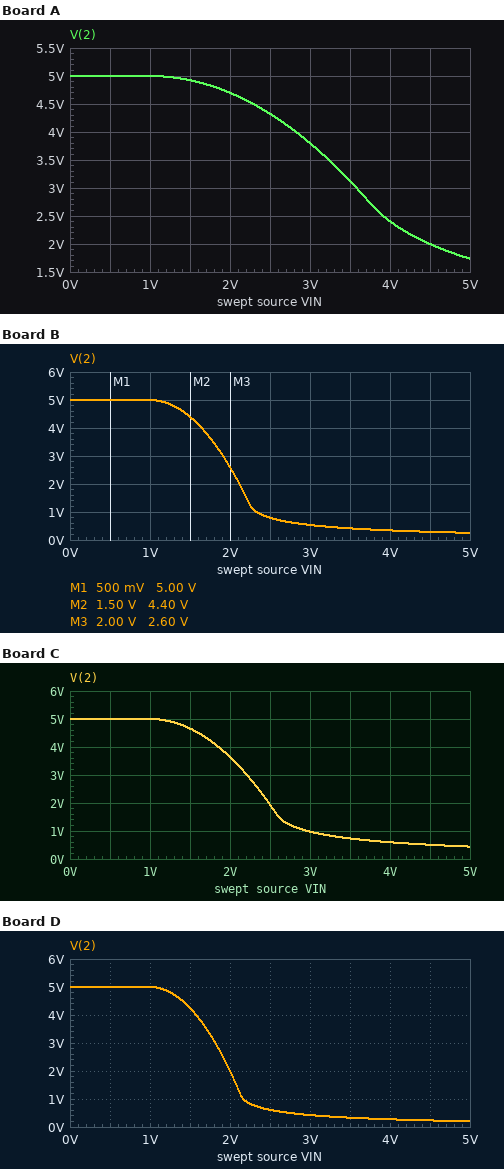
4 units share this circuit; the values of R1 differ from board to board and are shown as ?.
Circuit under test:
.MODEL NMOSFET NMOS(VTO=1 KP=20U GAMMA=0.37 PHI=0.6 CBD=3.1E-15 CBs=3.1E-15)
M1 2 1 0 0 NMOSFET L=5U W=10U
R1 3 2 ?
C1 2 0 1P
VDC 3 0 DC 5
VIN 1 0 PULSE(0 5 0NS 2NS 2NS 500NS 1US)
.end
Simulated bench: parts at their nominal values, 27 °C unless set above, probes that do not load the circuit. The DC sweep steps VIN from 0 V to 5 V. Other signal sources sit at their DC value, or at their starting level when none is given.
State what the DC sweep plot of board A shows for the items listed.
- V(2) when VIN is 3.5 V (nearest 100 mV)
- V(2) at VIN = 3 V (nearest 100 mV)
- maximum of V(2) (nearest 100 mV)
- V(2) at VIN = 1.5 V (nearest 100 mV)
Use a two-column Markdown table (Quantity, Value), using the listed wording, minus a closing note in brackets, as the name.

| Quantity | Value |
|---|---|
| V(2) when VIN is 3.5 V | 3.1 V |
| V(2) at VIN = 3 V | 3.8 V |
| maximum of V(2) | 5.0 V |
| V(2) at VIN = 1.5 V | 4.9 V |
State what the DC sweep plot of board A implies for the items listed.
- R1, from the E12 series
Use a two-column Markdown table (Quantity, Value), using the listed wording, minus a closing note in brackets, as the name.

| Quantity | Value |
|---|---|
| R1, from the E12 series | 15 kΩ |
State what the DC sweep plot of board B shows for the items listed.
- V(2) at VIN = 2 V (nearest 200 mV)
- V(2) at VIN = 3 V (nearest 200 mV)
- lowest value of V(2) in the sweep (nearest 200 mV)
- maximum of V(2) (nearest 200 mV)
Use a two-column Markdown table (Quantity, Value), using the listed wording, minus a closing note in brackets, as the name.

| Quantity | Value |
|---|---|
| V(2) at VIN = 2 V | 2.6 V |
| V(2) at VIN = 3 V | 600 mV |
| lowest value of V(2) in the sweep | 200 mV |
| maximum of V(2) | 5.0 V |
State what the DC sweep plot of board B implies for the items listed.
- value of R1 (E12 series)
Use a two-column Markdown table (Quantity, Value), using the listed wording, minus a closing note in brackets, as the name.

| Quantity | Value |
|---|---|
| value of R1 | 120 kΩ |
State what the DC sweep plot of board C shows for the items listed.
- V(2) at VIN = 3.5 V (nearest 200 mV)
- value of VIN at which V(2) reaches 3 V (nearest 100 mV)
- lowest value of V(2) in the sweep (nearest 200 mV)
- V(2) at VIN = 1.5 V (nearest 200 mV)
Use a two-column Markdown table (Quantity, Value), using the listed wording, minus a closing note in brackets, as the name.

| Quantity | Value |
|---|---|
| V(2) at VIN = 3.5 V | 800 mV |
| value of VIN at which V(2) reaches 3 V | 2.2 V |
| lowest value of V(2) in the sweep | 400 mV |
| V(2) at VIN = 1.5 V | 4.6 V |
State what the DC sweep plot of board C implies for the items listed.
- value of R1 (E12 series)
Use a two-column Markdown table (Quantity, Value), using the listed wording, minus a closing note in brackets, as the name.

| Quantity | Value |
|---|---|
| value of R1 | 68 kΩ |
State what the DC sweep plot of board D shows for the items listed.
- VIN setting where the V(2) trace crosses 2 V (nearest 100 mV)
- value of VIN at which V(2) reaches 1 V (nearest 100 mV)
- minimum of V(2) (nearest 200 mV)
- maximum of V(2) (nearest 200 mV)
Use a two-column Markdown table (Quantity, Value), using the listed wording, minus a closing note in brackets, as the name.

| Quantity | Value |
|---|---|
| VIN setting where the V(2) trace crosses 2 V | 2.0 V |
| value of VIN at which V(2) reaches 1 V | 2.2 V |
| minimum of V(2) | 200 mV |
| maximum of V(2) | 5.0 V |
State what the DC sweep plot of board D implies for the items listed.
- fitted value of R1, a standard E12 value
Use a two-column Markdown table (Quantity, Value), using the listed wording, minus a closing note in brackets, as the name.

| Quantity | Value |
|---|---|
| fitted value of R1, a standard E12 value | 150 kΩ |
